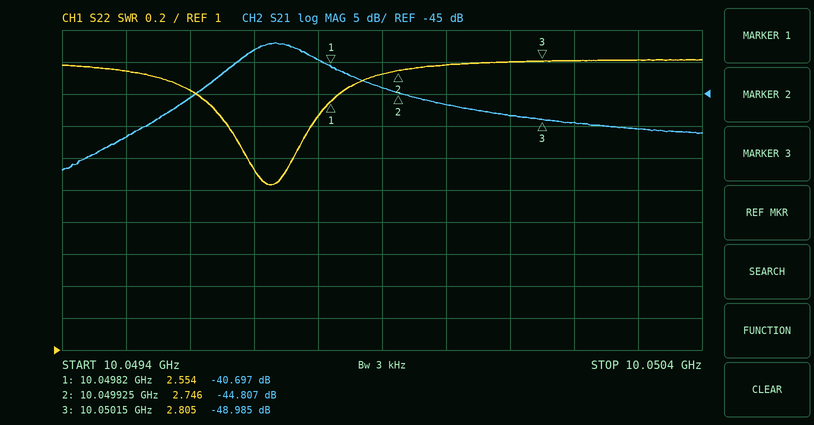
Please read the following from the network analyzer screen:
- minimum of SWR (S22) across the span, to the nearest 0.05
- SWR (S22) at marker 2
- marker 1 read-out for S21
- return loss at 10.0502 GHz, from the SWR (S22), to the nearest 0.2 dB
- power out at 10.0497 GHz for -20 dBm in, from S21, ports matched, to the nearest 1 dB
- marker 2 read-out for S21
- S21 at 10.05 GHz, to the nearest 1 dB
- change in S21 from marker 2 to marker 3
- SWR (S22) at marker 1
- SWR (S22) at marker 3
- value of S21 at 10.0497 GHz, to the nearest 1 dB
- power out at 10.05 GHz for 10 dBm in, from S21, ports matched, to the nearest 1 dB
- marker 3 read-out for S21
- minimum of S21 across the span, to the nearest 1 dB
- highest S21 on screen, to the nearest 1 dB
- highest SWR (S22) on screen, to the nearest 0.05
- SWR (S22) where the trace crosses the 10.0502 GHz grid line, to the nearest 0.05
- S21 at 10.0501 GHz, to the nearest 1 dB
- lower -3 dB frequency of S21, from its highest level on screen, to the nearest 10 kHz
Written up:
2.05
2.746
-40.697 dB
6.4 dB
-58 dBm
-44.807 dB
-47 dB
-4.178 dB
2.554
2.805
-38 dB
-37 dBm
-48.985 dB
-57 dB
-37 dB
2.80
2.80
-48 dB
10.04967 GHz
